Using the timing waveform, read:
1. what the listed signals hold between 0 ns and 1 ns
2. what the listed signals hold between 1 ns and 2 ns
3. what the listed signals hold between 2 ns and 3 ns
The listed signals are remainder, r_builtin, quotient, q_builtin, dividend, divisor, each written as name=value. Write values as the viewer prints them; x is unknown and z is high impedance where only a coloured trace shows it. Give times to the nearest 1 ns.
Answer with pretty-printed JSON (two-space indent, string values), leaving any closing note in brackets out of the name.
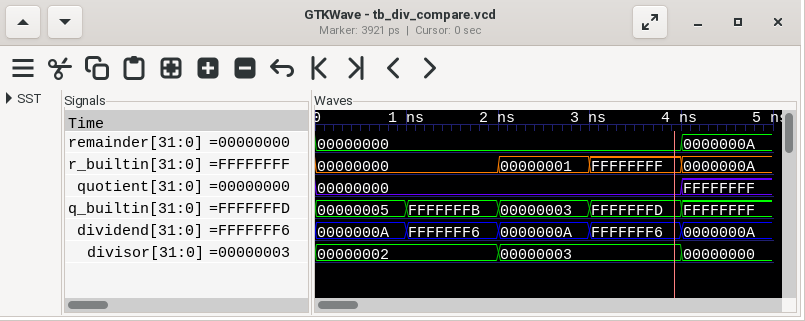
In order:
{
  "what the listed signals hold between 0 ns and 1 ns": "remainder=00000000, r_builtin=00000000, quotient=00000000, q_builtin=00000005, dividend=0000000A, divisor=00000002",
  "what the listed signals hold between 1 ns and 2 ns": "remainder=00000000, r_builtin=00000000, quotient=00000000, q_builtin=FFFFFFFB, dividend=FFFFFFF6, divisor=00000002",
  "what the listed signals hold between 2 ns and 3 ns": "remainder=00000000, r_builtin=00000001, quotient=00000000, q_builtin=00000003, dividend=0000000A, divisor=00000003"
}
